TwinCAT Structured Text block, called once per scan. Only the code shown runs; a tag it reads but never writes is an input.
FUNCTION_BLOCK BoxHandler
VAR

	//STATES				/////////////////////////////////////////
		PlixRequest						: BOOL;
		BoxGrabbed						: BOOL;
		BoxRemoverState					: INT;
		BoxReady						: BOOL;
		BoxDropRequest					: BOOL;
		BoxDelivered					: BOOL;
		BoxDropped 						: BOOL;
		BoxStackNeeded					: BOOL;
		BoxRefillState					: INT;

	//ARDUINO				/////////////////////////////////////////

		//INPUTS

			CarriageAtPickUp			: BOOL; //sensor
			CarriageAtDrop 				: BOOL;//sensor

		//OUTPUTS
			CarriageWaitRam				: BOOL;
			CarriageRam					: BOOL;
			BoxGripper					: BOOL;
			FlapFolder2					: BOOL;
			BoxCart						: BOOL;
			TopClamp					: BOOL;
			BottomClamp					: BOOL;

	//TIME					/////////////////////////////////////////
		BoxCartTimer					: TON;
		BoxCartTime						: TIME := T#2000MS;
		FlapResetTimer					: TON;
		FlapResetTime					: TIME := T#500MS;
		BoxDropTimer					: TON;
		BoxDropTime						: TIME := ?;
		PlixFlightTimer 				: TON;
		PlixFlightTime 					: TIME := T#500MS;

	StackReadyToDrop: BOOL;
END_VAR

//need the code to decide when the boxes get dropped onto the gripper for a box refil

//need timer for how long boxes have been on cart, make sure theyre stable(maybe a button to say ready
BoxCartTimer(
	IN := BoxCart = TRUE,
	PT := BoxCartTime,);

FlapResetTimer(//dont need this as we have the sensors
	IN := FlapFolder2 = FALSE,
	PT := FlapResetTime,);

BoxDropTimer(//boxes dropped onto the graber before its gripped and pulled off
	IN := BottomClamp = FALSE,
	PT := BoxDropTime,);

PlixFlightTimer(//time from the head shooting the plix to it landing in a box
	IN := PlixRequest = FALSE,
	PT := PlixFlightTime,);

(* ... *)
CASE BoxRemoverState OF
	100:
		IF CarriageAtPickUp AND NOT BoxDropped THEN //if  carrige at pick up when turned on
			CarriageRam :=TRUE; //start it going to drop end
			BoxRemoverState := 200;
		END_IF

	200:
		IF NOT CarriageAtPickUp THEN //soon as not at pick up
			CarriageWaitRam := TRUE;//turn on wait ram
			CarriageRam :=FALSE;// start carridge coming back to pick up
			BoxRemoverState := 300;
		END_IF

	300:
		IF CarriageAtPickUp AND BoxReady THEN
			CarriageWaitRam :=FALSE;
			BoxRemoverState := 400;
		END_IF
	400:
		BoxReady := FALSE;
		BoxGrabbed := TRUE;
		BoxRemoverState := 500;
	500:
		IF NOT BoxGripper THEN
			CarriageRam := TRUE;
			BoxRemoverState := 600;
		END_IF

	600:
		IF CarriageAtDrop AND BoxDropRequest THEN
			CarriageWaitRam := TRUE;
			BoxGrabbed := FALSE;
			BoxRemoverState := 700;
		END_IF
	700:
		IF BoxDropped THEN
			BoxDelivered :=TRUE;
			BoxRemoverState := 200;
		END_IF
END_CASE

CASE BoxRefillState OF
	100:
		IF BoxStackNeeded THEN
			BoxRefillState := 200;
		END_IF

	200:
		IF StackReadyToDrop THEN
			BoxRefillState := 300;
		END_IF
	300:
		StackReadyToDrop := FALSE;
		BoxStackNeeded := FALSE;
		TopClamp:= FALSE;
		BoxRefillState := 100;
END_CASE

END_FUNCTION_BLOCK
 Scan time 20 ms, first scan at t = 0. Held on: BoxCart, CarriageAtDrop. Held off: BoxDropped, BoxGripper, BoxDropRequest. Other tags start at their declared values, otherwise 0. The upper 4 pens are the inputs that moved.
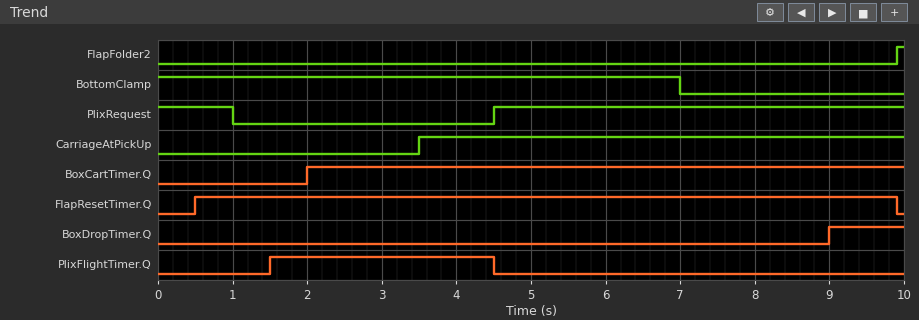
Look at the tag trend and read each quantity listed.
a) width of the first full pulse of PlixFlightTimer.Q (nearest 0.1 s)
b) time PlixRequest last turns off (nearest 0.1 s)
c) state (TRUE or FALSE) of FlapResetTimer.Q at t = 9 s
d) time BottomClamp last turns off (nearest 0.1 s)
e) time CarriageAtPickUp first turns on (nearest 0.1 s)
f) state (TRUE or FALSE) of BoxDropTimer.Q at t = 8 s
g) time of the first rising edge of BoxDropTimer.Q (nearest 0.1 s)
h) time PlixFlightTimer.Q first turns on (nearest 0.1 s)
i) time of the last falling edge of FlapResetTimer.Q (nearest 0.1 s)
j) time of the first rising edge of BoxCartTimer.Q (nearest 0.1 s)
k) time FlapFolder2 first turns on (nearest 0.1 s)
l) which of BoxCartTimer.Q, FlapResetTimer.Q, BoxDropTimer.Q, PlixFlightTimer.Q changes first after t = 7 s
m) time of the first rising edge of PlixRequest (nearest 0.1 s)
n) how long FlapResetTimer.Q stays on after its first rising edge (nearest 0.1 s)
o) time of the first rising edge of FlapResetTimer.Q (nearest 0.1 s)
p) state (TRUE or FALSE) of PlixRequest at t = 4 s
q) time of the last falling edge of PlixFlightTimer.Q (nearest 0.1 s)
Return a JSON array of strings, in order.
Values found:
["3.0 s", "1.0 s", "TRUE", "7.0 s", "3.5 s", "FALSE", "9.0 s", "1.5 s", "9.9 s", "2.0 s", "9.9 s", "BoxDropTimer.Q", "4.5 s", "9.4 s", "0.5 s", "FALSE", "4.5 s"]
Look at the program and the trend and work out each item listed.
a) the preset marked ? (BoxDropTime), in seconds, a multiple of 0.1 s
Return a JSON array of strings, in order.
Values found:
["2.0 s"]
